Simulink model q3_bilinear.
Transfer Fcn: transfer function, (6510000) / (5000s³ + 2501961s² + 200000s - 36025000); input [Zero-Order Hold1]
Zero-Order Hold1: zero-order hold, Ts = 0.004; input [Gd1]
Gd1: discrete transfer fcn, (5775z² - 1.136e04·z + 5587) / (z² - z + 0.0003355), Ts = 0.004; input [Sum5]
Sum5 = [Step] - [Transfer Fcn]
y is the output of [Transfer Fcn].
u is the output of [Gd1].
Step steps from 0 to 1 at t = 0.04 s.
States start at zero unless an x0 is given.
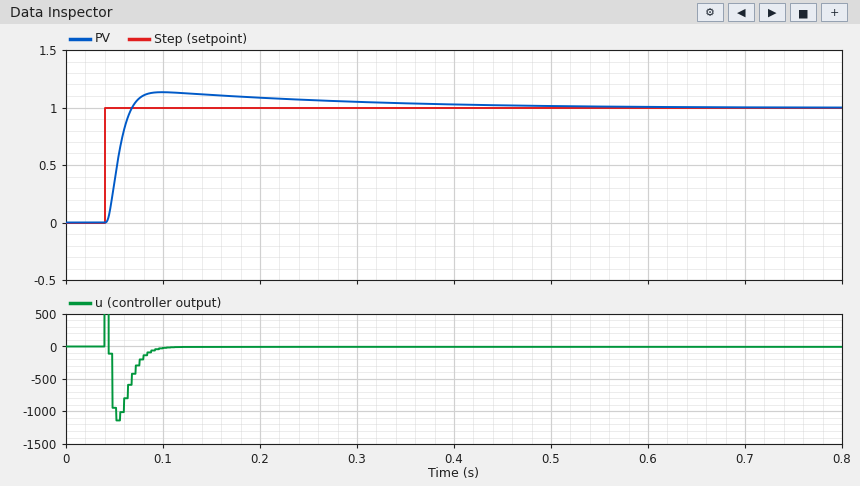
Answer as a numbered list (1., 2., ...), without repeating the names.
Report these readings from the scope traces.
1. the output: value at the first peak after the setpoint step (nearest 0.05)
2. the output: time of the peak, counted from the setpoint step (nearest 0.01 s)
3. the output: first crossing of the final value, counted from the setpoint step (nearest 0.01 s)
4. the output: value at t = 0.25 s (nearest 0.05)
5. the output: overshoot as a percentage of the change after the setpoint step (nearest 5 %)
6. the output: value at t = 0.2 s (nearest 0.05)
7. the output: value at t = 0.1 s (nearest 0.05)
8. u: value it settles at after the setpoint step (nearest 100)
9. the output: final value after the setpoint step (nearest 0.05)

1. 1.15
2. 0.06 s
3. 0.03 s
4. 1.05
5. 15 %
6. 1.10
7. 1.15
8. 0
9. 1.00
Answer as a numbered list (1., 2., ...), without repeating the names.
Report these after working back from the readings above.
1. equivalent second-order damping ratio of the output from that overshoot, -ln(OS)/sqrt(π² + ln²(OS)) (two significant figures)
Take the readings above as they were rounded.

1. 0.52
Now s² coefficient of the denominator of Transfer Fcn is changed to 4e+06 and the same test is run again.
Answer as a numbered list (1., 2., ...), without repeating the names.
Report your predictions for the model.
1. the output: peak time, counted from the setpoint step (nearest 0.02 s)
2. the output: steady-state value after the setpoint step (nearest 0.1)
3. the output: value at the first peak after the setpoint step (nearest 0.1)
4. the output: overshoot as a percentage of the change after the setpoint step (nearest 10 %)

1. 0.10 s
2. 1.0
3. 1.2
4. 20 %
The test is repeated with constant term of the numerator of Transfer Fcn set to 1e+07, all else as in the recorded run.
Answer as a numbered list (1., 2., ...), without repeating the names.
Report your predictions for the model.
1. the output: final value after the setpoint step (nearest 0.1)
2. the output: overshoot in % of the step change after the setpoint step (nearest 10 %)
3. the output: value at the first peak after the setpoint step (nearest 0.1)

1. 1.0
2. 20 %
3. 1.2
